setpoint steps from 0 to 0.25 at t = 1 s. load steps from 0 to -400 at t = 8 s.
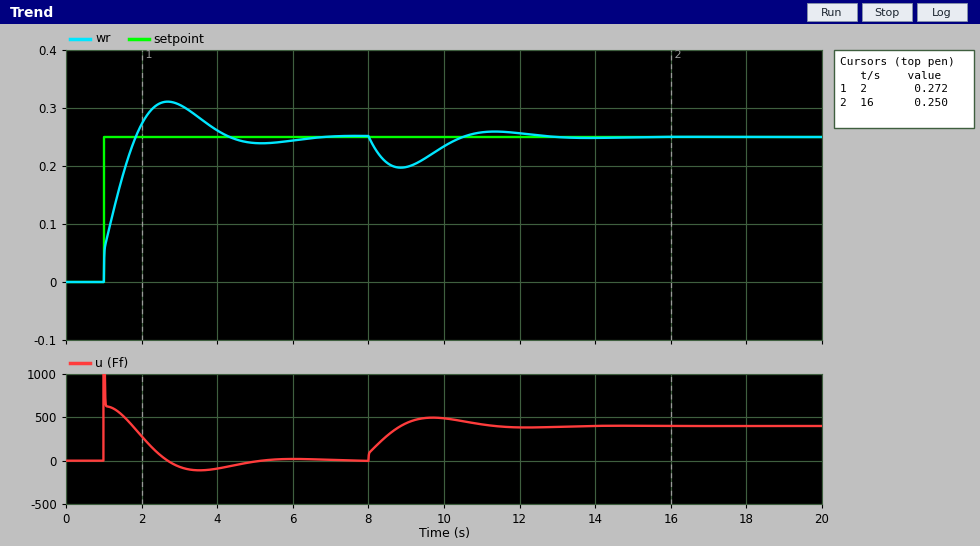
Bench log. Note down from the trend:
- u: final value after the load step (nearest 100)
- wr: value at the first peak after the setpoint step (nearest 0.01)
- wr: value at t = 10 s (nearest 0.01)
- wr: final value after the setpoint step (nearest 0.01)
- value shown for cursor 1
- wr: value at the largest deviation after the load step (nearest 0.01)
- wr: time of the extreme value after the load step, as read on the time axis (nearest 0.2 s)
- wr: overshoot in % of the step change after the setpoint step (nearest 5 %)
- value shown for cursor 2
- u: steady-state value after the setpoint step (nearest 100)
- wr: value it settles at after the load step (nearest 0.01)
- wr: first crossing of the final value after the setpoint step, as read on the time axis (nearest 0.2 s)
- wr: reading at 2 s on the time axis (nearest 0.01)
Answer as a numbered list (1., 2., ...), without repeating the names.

1. 400
2. 0.31
3. 0.23
4. 0.25
5. 0.272
6. 0.20
7. 8.8 s
8. 25 %
9. 0.250
10. 0
11. 0.25
12. 1.8 s
13. 0.27
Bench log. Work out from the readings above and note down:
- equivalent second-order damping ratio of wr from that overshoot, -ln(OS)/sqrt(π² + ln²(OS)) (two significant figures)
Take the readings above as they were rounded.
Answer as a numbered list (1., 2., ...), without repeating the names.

1. 0.40
